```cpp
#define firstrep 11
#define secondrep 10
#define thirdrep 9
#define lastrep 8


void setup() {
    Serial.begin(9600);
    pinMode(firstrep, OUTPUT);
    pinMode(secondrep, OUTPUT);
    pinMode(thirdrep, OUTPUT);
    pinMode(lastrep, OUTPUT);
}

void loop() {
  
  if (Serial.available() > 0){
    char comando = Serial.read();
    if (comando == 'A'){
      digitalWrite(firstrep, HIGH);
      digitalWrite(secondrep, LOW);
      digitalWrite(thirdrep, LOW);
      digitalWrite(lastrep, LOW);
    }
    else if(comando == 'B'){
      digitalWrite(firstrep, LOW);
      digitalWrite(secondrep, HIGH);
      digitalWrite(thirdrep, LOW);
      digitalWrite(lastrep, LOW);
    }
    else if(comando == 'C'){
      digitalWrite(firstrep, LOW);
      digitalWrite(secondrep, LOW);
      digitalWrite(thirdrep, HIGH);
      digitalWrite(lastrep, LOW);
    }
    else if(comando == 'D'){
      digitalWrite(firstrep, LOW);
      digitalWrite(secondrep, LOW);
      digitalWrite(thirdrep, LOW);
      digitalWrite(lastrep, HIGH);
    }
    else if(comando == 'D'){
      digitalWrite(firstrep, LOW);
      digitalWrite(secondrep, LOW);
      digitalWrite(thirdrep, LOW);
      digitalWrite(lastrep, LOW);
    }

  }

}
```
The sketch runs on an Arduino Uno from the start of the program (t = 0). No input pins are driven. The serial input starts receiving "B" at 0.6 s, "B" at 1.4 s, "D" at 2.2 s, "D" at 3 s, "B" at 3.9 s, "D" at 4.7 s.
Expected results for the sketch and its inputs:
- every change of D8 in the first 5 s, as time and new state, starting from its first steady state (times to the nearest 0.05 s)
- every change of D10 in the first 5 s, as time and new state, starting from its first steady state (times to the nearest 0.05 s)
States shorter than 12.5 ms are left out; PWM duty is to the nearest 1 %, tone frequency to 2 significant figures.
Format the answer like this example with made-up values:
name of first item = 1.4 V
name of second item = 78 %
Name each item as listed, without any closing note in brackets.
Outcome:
every change of D8 in the first 5 s, as time and new state, starting from its first steady state = 0 s low; 2.2 s high; 3.9 s low; 4.7 s high
every change of D10 in the first 5 s, as time and new state, starting from its first steady state = 0 s low; 0.6 s high; 2.2 s low; 3.9 s high; 4.7 s low
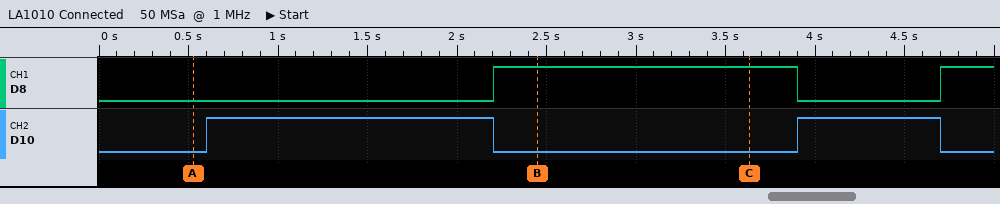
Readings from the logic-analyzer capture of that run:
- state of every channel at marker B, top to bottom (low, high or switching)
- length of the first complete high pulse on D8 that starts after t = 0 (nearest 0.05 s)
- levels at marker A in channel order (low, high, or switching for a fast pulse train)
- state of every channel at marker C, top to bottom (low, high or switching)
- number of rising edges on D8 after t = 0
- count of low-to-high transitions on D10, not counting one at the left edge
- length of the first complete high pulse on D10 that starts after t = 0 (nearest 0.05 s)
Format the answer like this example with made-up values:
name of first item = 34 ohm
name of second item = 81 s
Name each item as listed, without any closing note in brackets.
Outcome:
state of every channel at marker B, top to bottom = D8 high, D10 low
length of the first complete high pulse on D8 that starts after t = 0 = 1.70 s
levels at marker A in channel order = D8 low, D10 low
state of every channel at marker C, top to bottom = D8 high, D10 low
number of rising edges on D8 after t = 0 = 2
count of low-to-high transitions on D10, not counting one at the left edge = 2
length of the first complete high pulse on D10 that starts after t = 0 = 1.60 s
